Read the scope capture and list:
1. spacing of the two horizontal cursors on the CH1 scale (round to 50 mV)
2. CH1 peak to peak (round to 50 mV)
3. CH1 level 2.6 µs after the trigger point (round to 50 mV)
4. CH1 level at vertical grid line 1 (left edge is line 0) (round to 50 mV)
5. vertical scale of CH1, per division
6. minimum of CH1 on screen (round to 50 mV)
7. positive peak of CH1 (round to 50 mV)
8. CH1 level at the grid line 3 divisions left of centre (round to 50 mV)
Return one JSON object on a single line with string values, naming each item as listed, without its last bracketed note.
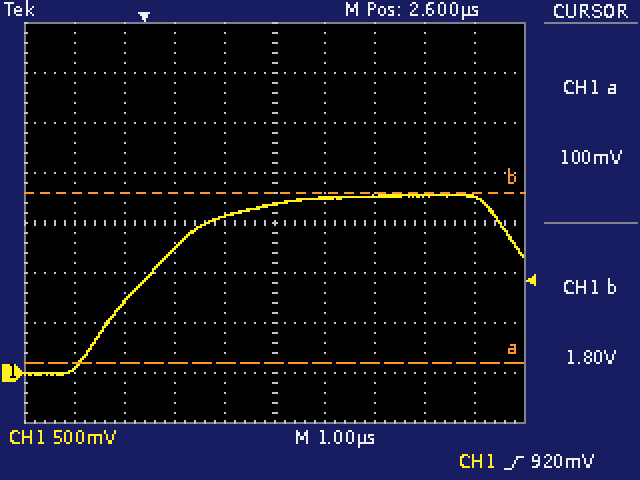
{"spacing of the two horizontal cursors on the CH1 scale": "1.70 V", "CH1 peak to peak": "1.80 V", "CH1 level 2.6 µs after the trigger point": "1.70 V", "CH1 level at vertical grid line 1 (left edge is line 0)": "50 mV", "vertical scale of CH1, per division": "500 mV", "minimum of CH1 on screen": "0 mV", "positive peak of CH1": "1.80 V", "CH1 level at the grid line 3 divisions left of centre": "700 mV"}
